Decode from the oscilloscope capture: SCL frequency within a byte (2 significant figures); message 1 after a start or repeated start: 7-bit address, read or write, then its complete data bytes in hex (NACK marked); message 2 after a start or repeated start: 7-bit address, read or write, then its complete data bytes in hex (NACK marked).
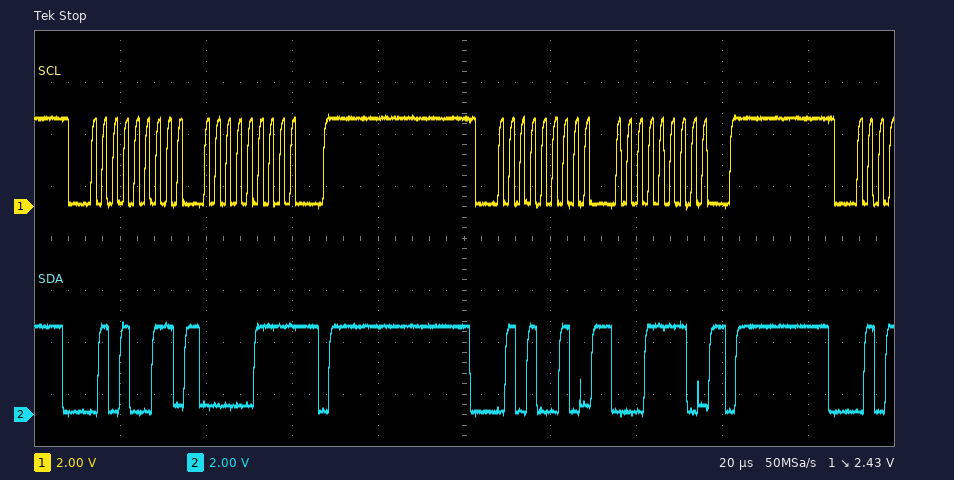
400 kHz
0x29 read: 07 NACK
0x29 write: 1E
